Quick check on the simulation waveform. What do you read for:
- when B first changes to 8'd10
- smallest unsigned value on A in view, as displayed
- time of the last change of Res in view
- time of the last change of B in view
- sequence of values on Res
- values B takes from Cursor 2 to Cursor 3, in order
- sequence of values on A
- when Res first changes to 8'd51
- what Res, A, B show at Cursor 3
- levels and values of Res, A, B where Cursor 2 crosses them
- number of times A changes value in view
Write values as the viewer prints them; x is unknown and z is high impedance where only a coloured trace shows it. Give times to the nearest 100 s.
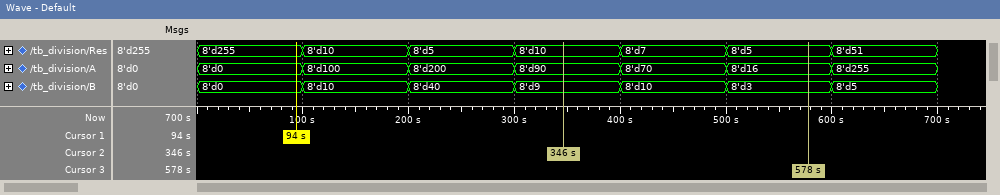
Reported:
100 s
8'd0
600 s
600 s
8'd255, 8'd10, 8'd5, 8'd10, 8'd7, 8'd5, 8'd51
8'd9, 8'd10, 8'd3
8'd0, 8'd100, 8'd200, 8'd90, 8'd70, 8'd16, 8'd255
600 s
Res=8'd5, A=8'd16, B=8'd3
Res=8'd10, A=8'd90, B=8'd9
6
